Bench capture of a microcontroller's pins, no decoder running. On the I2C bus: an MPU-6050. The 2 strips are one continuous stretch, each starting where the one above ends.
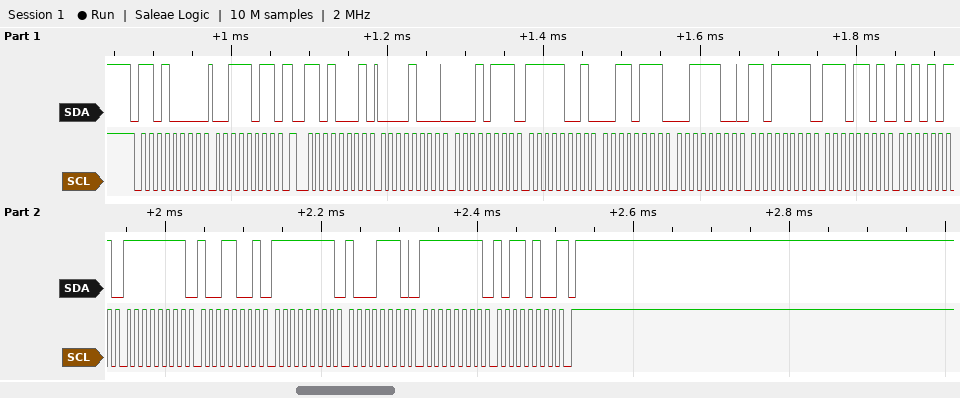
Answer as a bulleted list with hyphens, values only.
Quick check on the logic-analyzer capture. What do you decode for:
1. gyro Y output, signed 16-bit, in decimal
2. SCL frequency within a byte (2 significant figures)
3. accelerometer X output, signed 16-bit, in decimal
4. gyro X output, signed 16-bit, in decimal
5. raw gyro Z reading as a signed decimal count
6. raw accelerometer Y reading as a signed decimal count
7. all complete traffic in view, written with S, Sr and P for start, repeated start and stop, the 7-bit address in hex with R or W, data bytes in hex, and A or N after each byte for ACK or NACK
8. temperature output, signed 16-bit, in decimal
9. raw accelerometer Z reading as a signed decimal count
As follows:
- -114
- 100 kHz
- 2071
- -103
- -76
- -1737
- S 68W A 3B A Sr 68R A 08 A 17 A F9 A 37 A 3C A DF A ED A AB A FF A 99 A FF A 8E A FF A B4 N P
- -4693
- 15583
